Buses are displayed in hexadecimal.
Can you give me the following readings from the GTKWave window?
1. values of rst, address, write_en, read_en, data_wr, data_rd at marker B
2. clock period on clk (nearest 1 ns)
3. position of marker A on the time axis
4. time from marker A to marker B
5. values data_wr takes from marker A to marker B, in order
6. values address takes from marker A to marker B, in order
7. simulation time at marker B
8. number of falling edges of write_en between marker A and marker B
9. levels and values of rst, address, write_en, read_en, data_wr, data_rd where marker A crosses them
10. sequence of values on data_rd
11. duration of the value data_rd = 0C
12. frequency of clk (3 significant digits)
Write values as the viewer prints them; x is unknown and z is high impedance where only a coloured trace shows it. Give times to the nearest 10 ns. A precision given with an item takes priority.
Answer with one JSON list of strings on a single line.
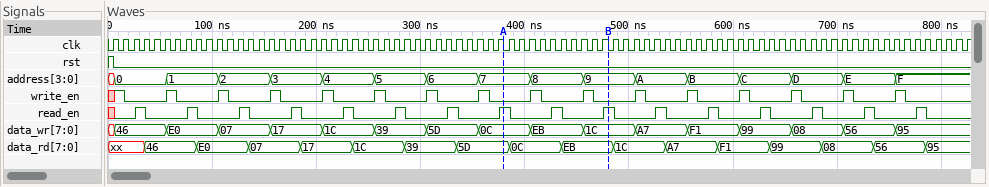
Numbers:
["rst=0, address=9, write_en=0, read_en=1, data_wr=1C, data_rd=EB", "10 ns", "380 ns", "100 ns", "0C, EB, 1C", "7, 8, 9", "480 ns", "2", "rst=0, address=7, write_en=0, read_en=1, data_wr=0C, data_rd=5D", "xx, 46, E0, 07, 17, 1C, 39, 5D, 0C, EB, 1C, A7, F1, 99, 08, 56, 95", "50 ns", "100 MHz"]
